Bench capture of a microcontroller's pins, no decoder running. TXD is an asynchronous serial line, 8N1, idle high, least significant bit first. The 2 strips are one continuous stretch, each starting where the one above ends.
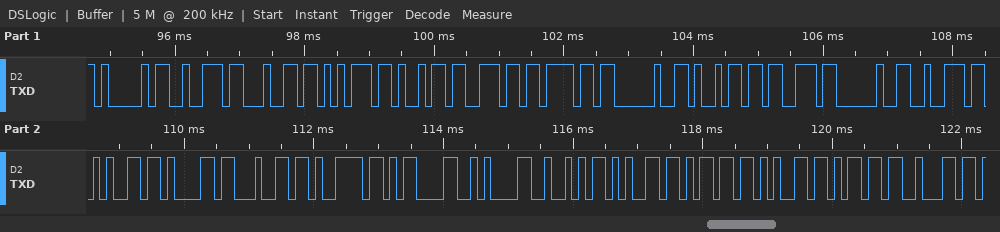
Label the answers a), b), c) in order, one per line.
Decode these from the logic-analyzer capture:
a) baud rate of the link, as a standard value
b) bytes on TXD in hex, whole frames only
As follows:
a) 9600 baud
b) 41 72 64 75 69 6E 6F 20 69 73 20 72 65 61 64 79 0D 0A 52 65 6D 65 6D 62
